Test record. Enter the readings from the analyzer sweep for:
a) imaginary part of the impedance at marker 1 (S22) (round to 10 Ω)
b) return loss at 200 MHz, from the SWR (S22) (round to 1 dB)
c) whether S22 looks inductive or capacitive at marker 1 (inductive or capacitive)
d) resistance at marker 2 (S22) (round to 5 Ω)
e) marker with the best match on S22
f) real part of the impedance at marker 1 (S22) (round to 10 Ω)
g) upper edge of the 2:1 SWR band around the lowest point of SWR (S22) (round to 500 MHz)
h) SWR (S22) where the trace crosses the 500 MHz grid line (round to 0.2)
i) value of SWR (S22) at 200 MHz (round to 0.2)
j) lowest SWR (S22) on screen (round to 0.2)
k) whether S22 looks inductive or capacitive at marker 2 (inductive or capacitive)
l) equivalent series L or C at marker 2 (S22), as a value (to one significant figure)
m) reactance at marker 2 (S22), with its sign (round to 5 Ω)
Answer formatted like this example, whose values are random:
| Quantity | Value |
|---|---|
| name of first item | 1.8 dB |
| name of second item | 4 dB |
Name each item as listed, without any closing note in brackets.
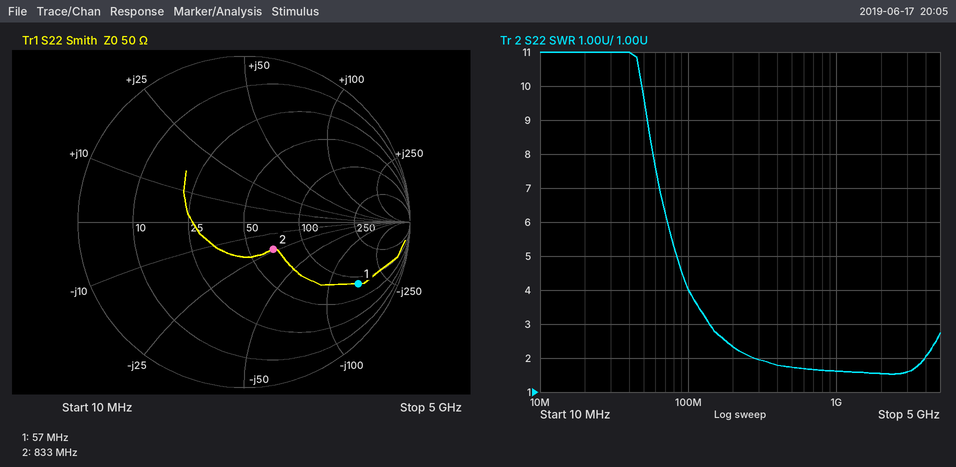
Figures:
| Quantity | Value |
|---|---|
| imaginary part of the impedance at marker 1 (S22) | -160 Ω |
| return loss at 200 MHz, from the SWR (S22) | 8 dB |
| whether S22 looks inductive or capacitive at marker 1 | capacitive |
| resistance at marker 2 (S22) | 65 Ω |
| marker with the best match on S22 | marker 2 |
| real part of the impedance at marker 1 (S22) | 80 Ω |
| upper edge of the 2:1 SWR band around the lowest point of SWR (S22) | 4.0 GHz |
| SWR (S22) where the trace crosses the 500 MHz grid line | 1.8 |
| value of SWR (S22) at 200 MHz | 2.4 |
| lowest SWR (S22) on screen | 1.6 |
| whether S22 looks inductive or capacitive at marker 2 | capacitive |
| equivalent series L or C at marker 2 (S22), as a value | 8 pF |
| reactance at marker 2 (S22), with its sign | -25 Ω |
